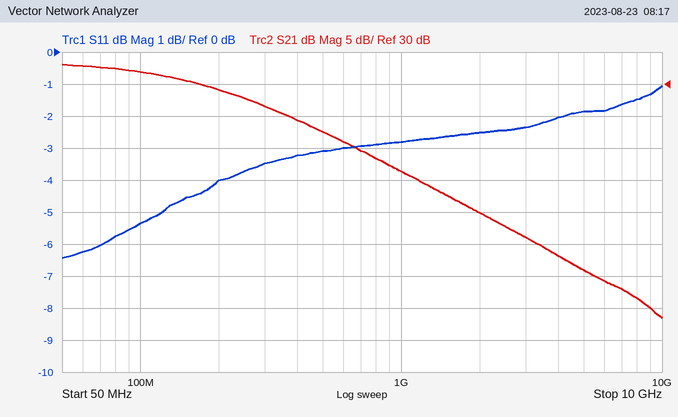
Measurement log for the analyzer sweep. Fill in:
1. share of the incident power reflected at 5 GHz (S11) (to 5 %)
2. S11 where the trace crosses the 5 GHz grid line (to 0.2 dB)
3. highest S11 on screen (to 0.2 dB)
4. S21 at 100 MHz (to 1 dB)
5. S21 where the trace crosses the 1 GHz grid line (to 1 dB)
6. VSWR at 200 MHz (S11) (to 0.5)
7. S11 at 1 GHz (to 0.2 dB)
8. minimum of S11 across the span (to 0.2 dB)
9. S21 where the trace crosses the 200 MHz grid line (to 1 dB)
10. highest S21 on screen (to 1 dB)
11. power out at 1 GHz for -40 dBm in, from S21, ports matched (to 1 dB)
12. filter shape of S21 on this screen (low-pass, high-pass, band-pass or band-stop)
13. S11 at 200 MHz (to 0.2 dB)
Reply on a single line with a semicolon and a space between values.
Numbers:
65 %; -1.8 dB; -1.0 dB; 32 dB; 16 dB; 4.5; -2.8 dB; -6.4 dB; 29 dB; 33 dB; -24 dBm; low-pass; -4.0 dB
